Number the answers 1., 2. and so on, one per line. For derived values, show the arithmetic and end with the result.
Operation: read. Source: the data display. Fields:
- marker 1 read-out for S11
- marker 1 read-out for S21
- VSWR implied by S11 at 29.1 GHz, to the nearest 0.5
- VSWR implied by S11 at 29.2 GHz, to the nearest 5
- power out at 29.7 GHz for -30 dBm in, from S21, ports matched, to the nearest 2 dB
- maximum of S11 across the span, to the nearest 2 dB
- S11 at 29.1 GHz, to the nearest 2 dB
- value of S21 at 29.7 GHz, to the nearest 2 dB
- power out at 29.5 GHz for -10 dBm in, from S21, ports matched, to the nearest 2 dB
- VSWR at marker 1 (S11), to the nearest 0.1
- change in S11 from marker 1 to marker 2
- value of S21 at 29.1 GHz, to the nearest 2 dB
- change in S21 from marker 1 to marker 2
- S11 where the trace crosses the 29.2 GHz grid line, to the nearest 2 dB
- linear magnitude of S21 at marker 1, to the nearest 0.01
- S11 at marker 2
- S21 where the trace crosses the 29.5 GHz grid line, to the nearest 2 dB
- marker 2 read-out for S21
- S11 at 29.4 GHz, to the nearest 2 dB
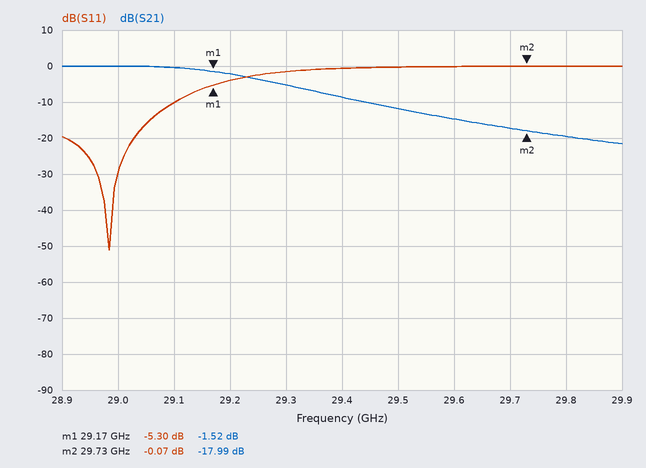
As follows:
1. -5.30 dB
2. -1.52 dB
3. |Γ| = 10^(-10/20) = 0.3162; VSWR = (1 + 0.3162)/(1 − 0.3162) ≈ 1.92, so 2.0 to the nearest 0.5
4. |Γ| = 10^(-4/20) = 0.6310; VSWR = (1 + 0.6310)/(1 − 0.6310) ≈ 4.42, so 5 to the nearest 5
5. -30 dBm + (-18 dB) = -48 dBm
6. 0 dB
7. -10 dB
8. -18 dB
9. -10 dBm + (-12 dB) = -22 dBm
10. (1 + 0.5433)/(1 − 0.5433) ≈ 3.4
11. -0.07 − (-5.3) = 5.23 dB
12. 0 dB
13. -17.99 − (-1.52) = -16.47 dB
14. -4 dB
15. 10^(-1.52/20) ≈ 0.84
16. -0.07 dB
17. -12 dB
18. -17.99 dB
19. 0 dB
